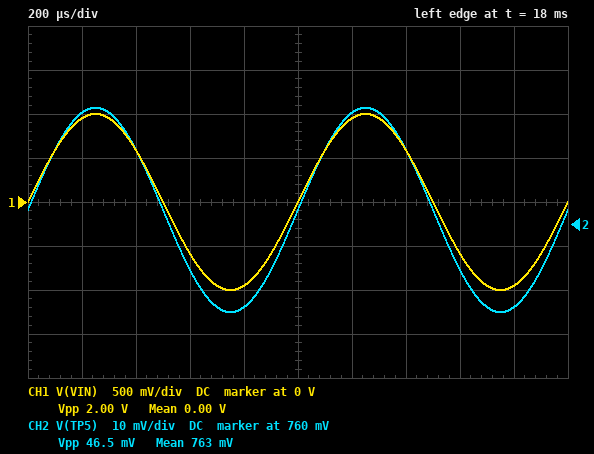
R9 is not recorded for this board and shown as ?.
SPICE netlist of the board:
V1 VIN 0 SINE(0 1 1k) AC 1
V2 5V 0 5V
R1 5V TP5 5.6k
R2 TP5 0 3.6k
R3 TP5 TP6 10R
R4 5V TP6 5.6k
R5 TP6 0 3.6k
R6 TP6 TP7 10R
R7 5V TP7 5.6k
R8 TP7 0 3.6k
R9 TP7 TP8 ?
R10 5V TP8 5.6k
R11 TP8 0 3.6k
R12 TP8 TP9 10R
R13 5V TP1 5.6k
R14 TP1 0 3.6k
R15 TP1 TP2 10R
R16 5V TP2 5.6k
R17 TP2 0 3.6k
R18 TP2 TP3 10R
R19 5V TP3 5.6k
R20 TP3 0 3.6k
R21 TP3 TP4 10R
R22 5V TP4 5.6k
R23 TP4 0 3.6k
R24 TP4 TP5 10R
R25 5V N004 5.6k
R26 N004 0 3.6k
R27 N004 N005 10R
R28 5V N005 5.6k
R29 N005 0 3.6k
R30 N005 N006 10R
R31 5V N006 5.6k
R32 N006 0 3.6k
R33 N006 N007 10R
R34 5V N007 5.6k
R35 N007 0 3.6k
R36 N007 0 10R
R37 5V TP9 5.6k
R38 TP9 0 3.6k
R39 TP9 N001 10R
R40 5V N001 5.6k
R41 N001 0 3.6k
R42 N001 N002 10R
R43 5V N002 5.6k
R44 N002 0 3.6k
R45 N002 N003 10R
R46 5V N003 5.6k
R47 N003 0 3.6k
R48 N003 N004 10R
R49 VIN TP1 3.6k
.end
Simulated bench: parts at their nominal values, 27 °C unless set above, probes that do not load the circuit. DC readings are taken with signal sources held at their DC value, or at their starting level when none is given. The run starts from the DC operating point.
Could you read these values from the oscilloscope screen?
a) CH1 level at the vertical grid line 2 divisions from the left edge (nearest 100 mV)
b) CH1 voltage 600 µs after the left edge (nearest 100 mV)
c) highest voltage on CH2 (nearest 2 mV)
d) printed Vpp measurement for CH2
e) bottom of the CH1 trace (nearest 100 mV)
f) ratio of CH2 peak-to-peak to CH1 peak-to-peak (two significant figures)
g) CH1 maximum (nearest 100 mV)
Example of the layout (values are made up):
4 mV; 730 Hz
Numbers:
600 mV; -600 mV; 786 mV; 46.5 mV; -1.0 V; 0.023; 1.0 V
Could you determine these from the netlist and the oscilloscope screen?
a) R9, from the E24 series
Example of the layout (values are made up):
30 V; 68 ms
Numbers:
24 Ω
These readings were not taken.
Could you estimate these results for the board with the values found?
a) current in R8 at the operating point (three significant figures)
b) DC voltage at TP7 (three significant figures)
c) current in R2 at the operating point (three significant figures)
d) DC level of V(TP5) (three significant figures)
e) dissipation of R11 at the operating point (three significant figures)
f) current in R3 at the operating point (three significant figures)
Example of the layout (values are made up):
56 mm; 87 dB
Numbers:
197 µA; 709 mV; 212 µA; 763 mV; 108 µW; 2.44 mA
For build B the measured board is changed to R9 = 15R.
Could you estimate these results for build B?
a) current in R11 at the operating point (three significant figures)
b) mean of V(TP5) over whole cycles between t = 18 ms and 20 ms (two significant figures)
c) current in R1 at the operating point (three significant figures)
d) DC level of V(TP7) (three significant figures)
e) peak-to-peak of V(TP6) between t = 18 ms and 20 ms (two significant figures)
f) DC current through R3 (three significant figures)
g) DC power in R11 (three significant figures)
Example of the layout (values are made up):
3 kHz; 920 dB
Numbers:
175 µA; 740 mV; 761 µA; 684 mV; 40 mV; 2.49 mA; 110 µW
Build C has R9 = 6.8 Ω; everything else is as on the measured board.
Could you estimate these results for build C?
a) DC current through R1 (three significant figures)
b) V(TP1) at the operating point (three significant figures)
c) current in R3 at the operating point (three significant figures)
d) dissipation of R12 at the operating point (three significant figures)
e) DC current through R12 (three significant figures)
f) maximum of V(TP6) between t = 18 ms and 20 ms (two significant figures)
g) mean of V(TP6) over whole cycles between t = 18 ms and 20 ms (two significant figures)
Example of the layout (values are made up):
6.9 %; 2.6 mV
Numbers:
765 µA; 764 mV; 2.55 mA; 187 µW; 4.32 mA; 710 mV; 690 mV
